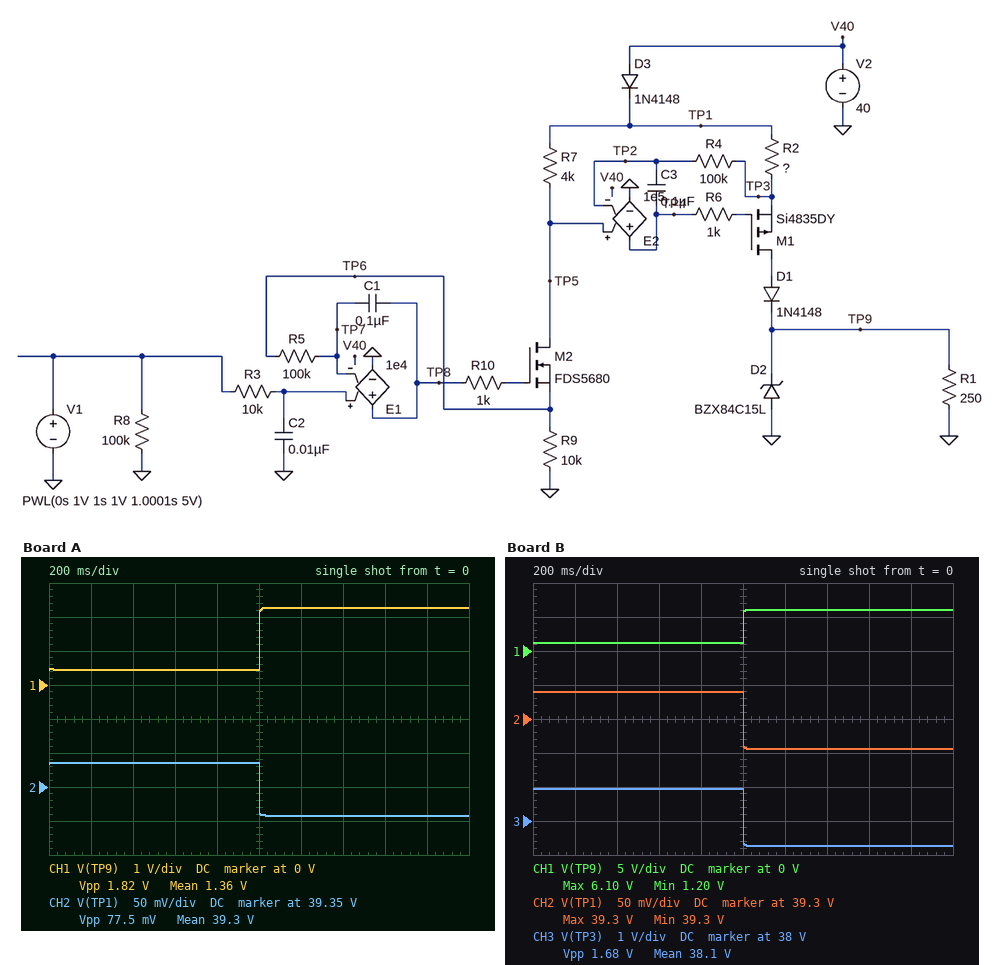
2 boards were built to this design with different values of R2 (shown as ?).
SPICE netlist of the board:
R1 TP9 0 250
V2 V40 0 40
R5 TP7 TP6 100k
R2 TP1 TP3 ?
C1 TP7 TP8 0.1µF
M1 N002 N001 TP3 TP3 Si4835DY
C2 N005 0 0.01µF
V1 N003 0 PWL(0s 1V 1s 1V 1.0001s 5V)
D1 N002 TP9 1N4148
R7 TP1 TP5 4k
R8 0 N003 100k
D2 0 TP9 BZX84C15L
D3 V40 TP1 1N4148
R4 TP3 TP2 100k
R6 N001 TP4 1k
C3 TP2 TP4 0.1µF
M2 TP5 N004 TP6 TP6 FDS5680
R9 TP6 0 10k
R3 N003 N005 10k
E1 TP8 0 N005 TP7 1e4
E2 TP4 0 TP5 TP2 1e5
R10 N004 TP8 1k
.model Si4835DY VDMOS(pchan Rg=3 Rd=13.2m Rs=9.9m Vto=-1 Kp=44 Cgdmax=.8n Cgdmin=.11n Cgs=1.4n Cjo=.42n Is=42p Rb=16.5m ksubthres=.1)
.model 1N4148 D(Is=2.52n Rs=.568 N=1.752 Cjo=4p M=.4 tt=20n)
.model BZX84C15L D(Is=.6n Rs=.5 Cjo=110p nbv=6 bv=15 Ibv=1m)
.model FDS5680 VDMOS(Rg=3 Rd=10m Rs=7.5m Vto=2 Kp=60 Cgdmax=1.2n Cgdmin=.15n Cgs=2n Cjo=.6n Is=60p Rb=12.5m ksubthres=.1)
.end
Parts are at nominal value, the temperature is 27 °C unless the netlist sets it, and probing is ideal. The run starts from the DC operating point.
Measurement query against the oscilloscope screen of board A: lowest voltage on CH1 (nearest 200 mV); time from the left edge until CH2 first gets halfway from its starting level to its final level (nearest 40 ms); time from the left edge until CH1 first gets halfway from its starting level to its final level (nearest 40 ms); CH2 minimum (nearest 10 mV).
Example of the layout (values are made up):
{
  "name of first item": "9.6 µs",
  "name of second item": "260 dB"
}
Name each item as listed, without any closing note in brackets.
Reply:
{
  "lowest voltage on CH1": "400 mV",
  "time from the left edge until CH2 first gets halfway from its starting level to its final level": "1.00 s",
  "time from the left edge until CH1 first gets halfway from its starting level to its final level": "1.00 s",
  "CH2 minimum": "39.31 V"
}
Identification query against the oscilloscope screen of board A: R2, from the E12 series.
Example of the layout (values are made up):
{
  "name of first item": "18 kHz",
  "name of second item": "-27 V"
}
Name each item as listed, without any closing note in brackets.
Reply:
{
  "R2, from the E12 series": "220 Ω"
}
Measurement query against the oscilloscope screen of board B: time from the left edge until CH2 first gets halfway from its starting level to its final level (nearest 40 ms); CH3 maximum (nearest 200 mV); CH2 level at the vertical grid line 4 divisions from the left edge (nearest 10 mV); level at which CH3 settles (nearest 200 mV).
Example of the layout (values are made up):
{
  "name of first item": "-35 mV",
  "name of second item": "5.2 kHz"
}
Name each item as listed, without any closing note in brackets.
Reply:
{
  "time from the left edge until CH2 first gets halfway from its starting level to its final level": "1.00 s",
  "CH3 maximum": "39.0 V",
  "CH2 level at the vertical grid line 4 divisions from the left edge": "39.34 V",
  "level at which CH3 settles": "37.2 V"
}
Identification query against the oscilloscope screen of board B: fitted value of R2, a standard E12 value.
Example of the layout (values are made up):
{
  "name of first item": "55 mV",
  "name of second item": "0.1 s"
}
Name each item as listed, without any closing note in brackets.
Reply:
{
  "fitted value of R2, a standard E12 value": "82 Ω"
}
